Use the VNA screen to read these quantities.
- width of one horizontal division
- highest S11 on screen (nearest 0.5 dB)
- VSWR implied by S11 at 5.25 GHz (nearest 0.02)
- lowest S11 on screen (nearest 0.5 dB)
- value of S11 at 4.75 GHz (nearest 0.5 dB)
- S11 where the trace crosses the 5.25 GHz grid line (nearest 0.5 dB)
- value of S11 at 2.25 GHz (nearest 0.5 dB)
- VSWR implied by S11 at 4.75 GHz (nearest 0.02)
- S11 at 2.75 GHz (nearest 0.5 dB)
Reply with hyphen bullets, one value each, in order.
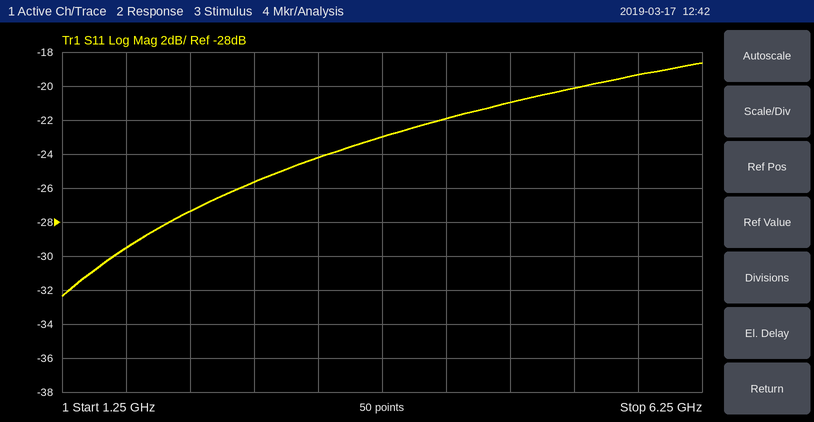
- 500 MHz
- -18.5 dB
- 1.22
- -32.5 dB
- -21.0 dB
- -20.0 dB
- -27.5 dB
- 1.20
- -25.5 dB
